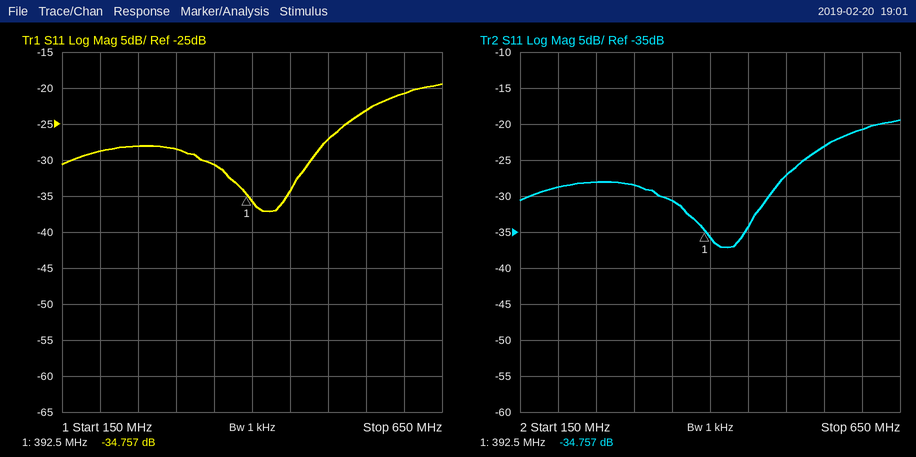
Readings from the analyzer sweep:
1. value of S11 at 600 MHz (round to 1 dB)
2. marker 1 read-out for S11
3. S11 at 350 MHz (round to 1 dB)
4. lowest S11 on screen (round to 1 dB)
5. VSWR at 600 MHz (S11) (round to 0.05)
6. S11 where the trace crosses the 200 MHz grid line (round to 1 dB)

-21 dB
-34.757 dB
-31 dB
-37 dB
1.20
-29 dB
